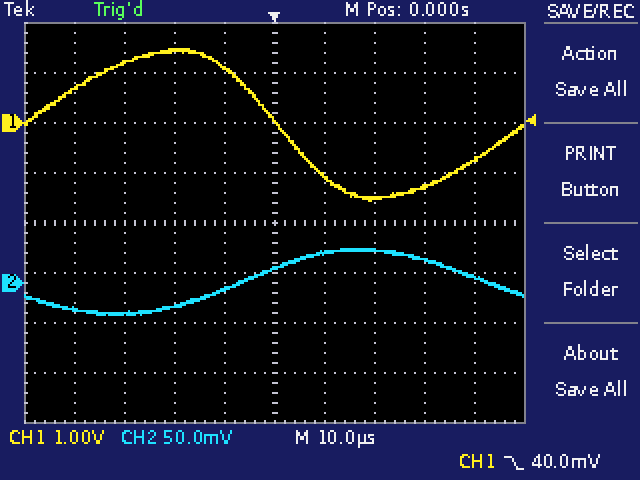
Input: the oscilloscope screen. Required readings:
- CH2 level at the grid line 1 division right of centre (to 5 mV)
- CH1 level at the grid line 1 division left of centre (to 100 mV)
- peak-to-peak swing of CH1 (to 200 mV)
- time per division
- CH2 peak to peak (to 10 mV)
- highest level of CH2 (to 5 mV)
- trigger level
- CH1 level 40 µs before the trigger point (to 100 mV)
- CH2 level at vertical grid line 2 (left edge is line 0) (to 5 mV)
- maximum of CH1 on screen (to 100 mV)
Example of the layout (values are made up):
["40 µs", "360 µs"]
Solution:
["30 mV", "1.1 V", "3.0 V", "10 µs", "70 mV", "35 mV", "40.0 mV", "700 mV", "-30 mV", "1.5 V"]
